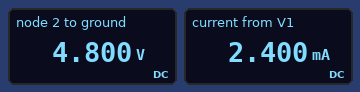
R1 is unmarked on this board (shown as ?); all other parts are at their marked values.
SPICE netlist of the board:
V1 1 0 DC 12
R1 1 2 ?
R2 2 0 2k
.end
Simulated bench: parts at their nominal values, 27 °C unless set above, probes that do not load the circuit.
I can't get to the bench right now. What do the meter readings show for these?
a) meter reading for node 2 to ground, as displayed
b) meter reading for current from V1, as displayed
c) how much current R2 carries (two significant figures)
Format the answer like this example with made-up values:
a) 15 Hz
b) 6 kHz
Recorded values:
a) 4.800 V
b) 2.400 mA
c) 2.4 mA
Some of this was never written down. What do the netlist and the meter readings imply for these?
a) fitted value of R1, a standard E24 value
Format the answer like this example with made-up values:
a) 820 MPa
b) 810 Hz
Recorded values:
a) 3 kΩ
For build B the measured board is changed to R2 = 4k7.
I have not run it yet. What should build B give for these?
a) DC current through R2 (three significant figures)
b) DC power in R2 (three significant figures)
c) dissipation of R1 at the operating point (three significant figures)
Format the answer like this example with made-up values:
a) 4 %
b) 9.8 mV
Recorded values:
a) 1.56 mA
b) 11.4 mW
c) 7.29 mW
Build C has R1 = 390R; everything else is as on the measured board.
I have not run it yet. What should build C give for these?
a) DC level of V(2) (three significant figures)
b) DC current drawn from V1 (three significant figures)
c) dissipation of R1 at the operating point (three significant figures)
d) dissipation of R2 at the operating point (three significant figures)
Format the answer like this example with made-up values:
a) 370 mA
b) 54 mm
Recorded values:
a) 10.0 V
b) 5.02 mA
c) 9.83 mW
d) 50.4 mW
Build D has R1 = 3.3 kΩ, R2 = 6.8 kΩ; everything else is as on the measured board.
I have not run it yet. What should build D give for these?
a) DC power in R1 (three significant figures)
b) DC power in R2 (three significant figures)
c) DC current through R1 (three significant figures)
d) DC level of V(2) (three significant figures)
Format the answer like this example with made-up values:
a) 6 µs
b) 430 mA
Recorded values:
a) 4.66 mW
b) 9.60 mW
c) 1.19 mA
d) 8.08 V
